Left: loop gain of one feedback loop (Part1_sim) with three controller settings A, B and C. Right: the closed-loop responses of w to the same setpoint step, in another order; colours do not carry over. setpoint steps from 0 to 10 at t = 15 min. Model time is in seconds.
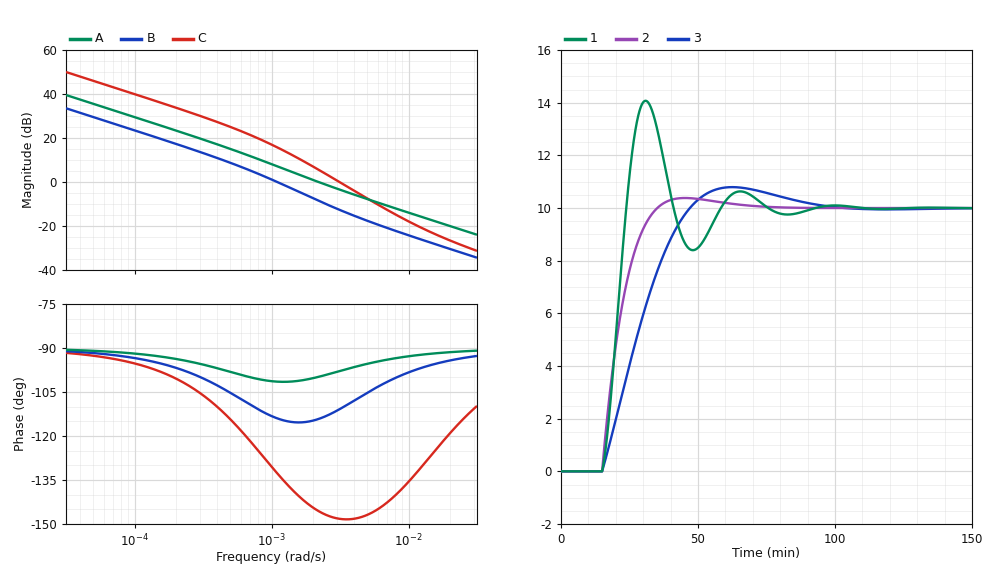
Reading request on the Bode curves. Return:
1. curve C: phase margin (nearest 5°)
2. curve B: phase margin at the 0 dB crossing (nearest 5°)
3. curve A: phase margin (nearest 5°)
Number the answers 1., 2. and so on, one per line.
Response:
1. 30°
2. 65°
3. 80°
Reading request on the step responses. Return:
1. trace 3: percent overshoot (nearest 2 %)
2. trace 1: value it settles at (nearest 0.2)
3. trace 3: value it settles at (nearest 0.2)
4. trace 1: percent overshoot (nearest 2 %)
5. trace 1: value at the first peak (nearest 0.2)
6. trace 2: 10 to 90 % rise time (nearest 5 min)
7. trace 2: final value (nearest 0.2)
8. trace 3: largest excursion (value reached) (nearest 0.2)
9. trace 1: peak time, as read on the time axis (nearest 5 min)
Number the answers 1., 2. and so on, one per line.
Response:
1. 8 %
2. 10.0
3. 10.0
4. 40 %
5. 14.0
6. 15 min
7. 10.0
8. 10.8
9. 30 min
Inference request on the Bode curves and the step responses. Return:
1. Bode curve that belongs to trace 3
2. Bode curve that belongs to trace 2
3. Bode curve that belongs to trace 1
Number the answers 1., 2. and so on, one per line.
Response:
1. B
2. A
3. C
